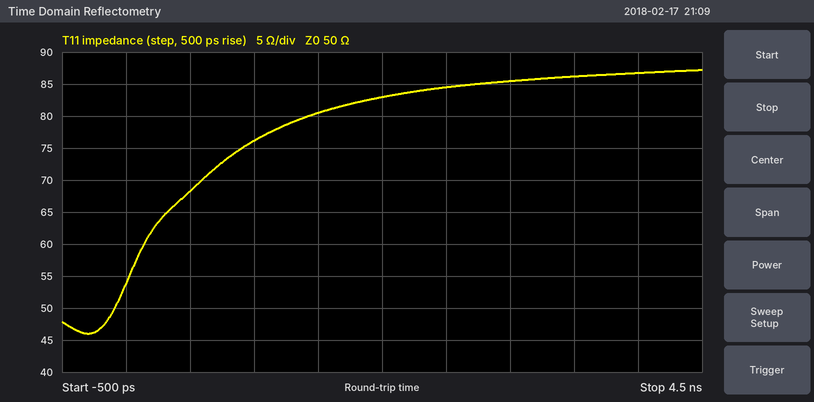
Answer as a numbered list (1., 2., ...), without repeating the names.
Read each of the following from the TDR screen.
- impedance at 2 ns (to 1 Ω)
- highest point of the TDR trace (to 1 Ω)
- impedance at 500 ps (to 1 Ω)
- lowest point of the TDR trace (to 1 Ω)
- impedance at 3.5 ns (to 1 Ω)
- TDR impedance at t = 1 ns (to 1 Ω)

1. 83 Ω
2. 87 Ω
3. 68 Ω
4. 46 Ω
5. 86 Ω
6. 76 Ω
